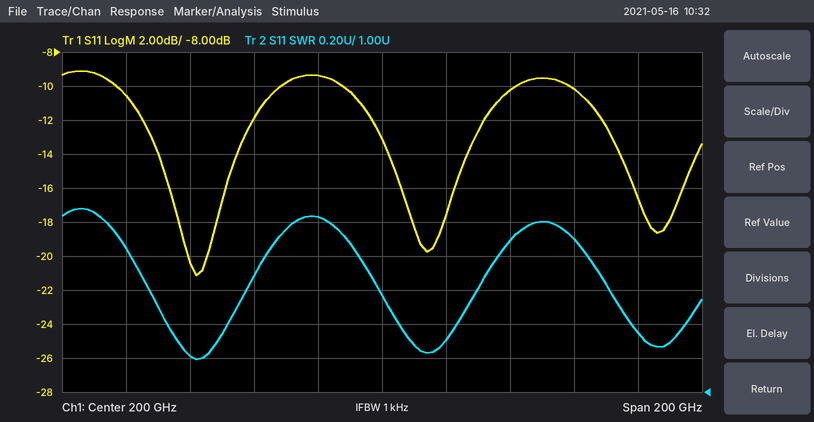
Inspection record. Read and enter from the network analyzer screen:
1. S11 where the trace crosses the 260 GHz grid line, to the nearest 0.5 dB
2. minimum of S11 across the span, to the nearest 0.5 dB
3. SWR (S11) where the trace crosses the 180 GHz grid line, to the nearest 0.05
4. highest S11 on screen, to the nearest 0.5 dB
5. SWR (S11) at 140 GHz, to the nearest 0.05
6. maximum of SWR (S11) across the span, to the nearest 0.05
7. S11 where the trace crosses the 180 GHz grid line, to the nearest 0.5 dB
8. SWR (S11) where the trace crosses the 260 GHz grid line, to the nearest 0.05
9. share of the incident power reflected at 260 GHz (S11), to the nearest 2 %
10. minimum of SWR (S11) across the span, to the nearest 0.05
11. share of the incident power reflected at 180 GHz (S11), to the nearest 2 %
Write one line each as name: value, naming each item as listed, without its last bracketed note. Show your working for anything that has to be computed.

S11 where the trace crosses the 260 GHz grid line, to the nearest 0.5 dB: -10.0 dB
minimum of S11 across the span, to the nearest 0.5 dB: -21.0 dB
SWR (S11) where the trace crosses the 180 GHz grid line, to the nearest 0.05: 2.05
highest S11 on screen, to the nearest 0.5 dB: -9.0 dB
SWR (S11) at 140 GHz, to the nearest 0.05: 1.20
maximum of SWR (S11) across the span, to the nearest 0.05: 2.10
S11 where the trace crosses the 180 GHz grid line, to the nearest 0.5 dB: -9.5 dB
SWR (S11) where the trace crosses the 260 GHz grid line, to the nearest 0.05: 1.90
share of the incident power reflected at 260 GHz (S11), to the nearest 2 %: 10^(-10/10) ≈ 10 %
minimum of SWR (S11) across the span, to the nearest 0.05: 1.20
share of the incident power reflected at 180 GHz (S11), to the nearest 2 %: 10^(-9.5/10) ≈ 11.2 %, so 12 % to the nearest 2 %
